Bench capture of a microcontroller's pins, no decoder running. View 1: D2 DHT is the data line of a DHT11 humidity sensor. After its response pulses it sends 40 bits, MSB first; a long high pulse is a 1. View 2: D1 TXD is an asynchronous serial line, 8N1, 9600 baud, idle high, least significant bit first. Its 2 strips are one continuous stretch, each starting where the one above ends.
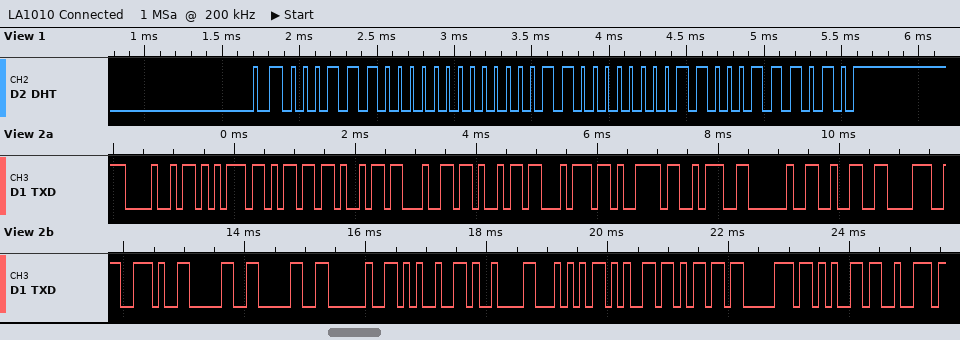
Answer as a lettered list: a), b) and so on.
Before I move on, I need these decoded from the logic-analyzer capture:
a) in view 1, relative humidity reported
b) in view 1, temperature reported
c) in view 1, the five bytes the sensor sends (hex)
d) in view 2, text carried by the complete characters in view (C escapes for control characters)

a) 28 %
b) 24.6 °C
c) 1C 00 18 06 3A
d) "Humidity: 28.00 %\tTemper"
